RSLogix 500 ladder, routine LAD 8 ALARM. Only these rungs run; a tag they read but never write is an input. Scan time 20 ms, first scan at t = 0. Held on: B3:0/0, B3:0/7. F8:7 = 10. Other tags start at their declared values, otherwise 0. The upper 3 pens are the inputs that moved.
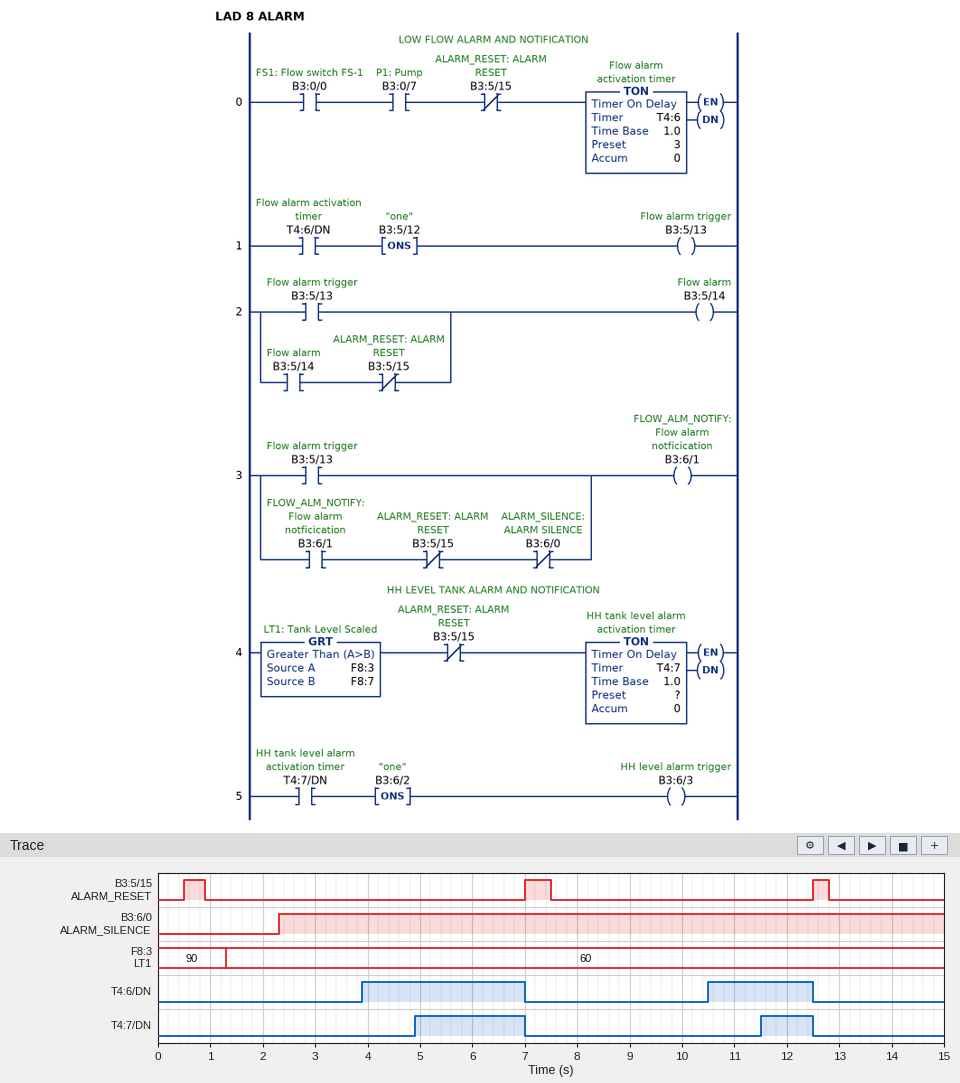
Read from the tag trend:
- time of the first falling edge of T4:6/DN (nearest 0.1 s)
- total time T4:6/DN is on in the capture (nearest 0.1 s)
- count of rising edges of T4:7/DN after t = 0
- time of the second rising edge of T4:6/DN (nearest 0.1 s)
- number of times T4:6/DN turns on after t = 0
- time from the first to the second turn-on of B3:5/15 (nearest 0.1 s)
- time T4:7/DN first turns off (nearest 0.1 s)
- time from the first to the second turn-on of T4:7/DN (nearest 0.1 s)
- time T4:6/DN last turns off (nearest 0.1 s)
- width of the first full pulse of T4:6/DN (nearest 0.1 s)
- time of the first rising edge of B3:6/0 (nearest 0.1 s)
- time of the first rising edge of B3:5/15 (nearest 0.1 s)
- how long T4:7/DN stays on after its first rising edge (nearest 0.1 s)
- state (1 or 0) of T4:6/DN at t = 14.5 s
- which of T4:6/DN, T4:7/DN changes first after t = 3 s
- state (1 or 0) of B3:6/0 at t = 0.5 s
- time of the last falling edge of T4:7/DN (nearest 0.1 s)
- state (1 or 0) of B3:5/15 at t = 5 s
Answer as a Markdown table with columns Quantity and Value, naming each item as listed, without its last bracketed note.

| Quantity | Value |
|---|---|
| time of the first falling edge of T4:6/DN | 7.0 s |
| total time T4:6/DN is on in the capture | 5.1 s |
| count of rising edges of T4:7/DN after t = 0 | 2 |
| time of the second rising edge of T4:6/DN | 10.5 s |
| number of times T4:6/DN turns on after t = 0 | 2 |
| time from the first to the second turn-on of B3:5/15 | 6.5 s |
| time T4:7/DN first turns off | 7.0 s |
| time from the first to the second turn-on of T4:7/DN | 6.6 s |
| time T4:6/DN last turns off | 12.5 s |
| width of the first full pulse of T4:6/DN | 3.1 s |
| time of the first rising edge of B3:6/0 | 2.3 s |
| time of the first rising edge of B3:5/15 | 0.5 s |
| how long T4:7/DN stays on after its first rising edge | 2.1 s |
| state (1 or 0) of T4:6/DN at t = 14.5 s | 0 |
| which of T4:6/DN, T4:7/DN changes first after t = 3 s | T4:6/DN |
| state (1 or 0) of B3:6/0 at t = 0.5 s | 0 |
| time of the last falling edge of T4:7/DN | 12.5 s |
| state (1 or 0) of B3:5/15 at t = 5 s | 0 |
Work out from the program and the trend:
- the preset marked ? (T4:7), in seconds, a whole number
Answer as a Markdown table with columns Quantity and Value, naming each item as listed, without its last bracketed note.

| Quantity | Value |
|---|---|
| the preset marked ? (T4:7), in seconds, a whole number | 4 s |
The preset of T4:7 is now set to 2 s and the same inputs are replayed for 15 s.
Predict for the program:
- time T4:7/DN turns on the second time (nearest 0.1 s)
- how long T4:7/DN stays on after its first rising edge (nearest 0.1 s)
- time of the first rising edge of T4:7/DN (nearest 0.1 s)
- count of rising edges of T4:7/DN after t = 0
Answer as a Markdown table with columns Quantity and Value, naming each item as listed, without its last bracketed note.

| Quantity | Value |
|---|---|
| time T4:7/DN turns on the second time | 9.5 s |
| how long T4:7/DN stays on after its first rising edge | 4.1 s |
| time of the first rising edge of T4:7/DN | 2.9 s |
| count of rising edges of T4:7/DN after t = 0 | 3 |
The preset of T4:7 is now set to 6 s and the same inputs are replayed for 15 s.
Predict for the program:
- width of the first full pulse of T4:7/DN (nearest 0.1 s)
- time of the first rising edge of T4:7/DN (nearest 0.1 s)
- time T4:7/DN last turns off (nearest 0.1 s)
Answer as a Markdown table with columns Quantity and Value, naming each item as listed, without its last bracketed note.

| Quantity | Value |
|---|---|
| width of the first full pulse of T4:7/DN | 0.1 s |
| time of the first rising edge of T4:7/DN | 6.9 s |
| time T4:7/DN last turns off | 7.0 s |
